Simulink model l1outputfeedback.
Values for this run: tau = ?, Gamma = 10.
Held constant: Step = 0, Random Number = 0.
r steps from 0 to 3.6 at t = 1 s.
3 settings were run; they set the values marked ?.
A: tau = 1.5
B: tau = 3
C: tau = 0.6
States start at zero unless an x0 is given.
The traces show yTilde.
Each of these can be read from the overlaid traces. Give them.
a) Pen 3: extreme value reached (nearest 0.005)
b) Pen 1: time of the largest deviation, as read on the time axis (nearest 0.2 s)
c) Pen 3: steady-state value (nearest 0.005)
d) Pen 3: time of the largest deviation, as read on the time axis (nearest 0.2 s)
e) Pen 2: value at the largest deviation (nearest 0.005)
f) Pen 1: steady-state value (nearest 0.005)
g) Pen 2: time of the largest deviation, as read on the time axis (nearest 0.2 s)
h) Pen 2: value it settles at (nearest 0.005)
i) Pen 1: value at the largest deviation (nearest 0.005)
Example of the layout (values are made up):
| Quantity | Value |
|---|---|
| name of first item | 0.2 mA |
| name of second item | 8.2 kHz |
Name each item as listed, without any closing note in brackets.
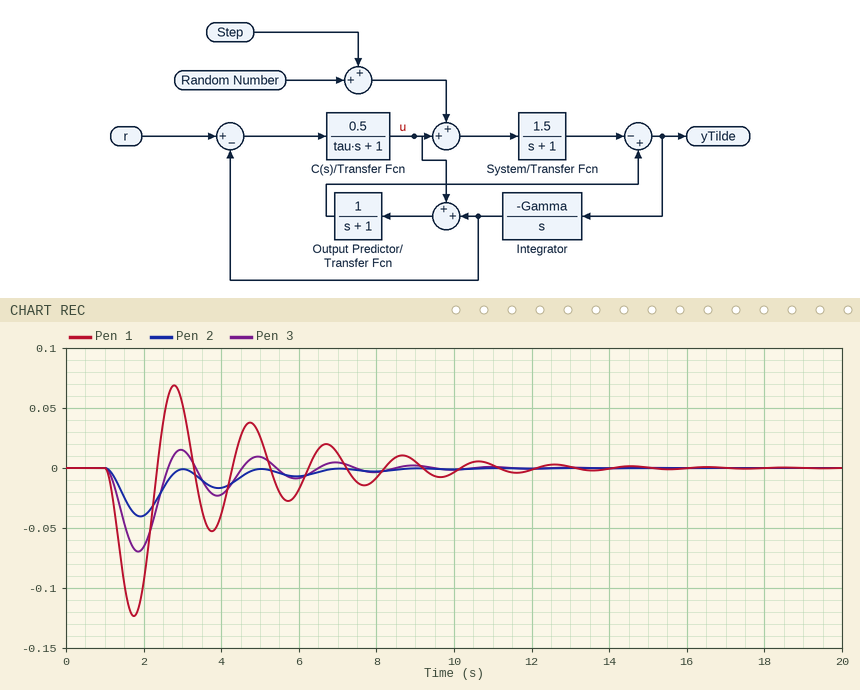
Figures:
| Quantity | Value |
|---|---|
| Pen 3: extreme value reached | -0.070 |
| Pen 1: time of the largest deviation, as read on the time axis | 1.8 s |
| Pen 3: steady-state value | 0.000 |
| Pen 3: time of the largest deviation, as read on the time axis | 1.8 s |
| Pen 2: value at the largest deviation | -0.040 |
| Pen 1: steady-state value | 0.000 |
| Pen 2: time of the largest deviation, as read on the time axis | 2.0 s |
| Pen 2: value it settles at | 0.000 |
| Pen 1: value at the largest deviation | -0.125 |
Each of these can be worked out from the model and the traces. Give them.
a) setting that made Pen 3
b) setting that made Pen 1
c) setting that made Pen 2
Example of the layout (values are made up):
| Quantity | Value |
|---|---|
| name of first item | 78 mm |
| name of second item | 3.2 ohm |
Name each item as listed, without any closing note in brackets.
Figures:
| Quantity | Value |
|---|---|
| setting that made Pen 3 | A |
| setting that made Pen 1 | C |
| setting that made Pen 2 | B |
